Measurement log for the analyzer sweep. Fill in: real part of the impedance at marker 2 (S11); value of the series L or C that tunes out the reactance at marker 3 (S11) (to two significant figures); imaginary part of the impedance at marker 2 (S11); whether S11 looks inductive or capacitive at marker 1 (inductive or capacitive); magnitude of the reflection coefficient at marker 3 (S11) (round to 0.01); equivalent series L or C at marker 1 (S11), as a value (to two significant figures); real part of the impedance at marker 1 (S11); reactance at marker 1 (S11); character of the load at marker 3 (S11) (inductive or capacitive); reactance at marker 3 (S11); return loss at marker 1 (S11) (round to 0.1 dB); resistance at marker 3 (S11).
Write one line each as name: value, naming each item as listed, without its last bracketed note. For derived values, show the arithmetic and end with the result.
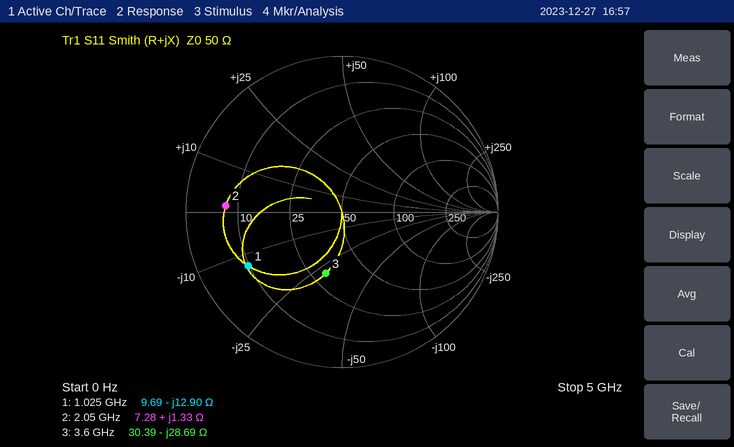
real part of the impedance at marker 2: 7.28 Ω
value of the series L or C that tunes out the reactance at marker 3 (S11): L = 28.69 Ω/(2π × 3.6 GHz) ≈ 1.3 nH
imaginary part of the impedance at marker 2: +1.33 Ω
whether S11 looks inductive or capacitive at marker 1: capacitive
magnitude of the reflection coefficient at marker 3 (S11): 0.41
equivalent series L or C at marker 1 (S11), as a value: C = 1/(2π × 1.025 GHz × 12.9 Ω) ≈ 12 pF
real part of the impedance at marker 1: 9.69 Ω
reactance at marker 1: -12.90 Ω
character of the load at marker 3 (S11): capacitive
reactance at marker 3: -28.69 Ω
return loss at marker 1 (S11): 3.2 dB
resistance at marker 3: 30.39 Ω
